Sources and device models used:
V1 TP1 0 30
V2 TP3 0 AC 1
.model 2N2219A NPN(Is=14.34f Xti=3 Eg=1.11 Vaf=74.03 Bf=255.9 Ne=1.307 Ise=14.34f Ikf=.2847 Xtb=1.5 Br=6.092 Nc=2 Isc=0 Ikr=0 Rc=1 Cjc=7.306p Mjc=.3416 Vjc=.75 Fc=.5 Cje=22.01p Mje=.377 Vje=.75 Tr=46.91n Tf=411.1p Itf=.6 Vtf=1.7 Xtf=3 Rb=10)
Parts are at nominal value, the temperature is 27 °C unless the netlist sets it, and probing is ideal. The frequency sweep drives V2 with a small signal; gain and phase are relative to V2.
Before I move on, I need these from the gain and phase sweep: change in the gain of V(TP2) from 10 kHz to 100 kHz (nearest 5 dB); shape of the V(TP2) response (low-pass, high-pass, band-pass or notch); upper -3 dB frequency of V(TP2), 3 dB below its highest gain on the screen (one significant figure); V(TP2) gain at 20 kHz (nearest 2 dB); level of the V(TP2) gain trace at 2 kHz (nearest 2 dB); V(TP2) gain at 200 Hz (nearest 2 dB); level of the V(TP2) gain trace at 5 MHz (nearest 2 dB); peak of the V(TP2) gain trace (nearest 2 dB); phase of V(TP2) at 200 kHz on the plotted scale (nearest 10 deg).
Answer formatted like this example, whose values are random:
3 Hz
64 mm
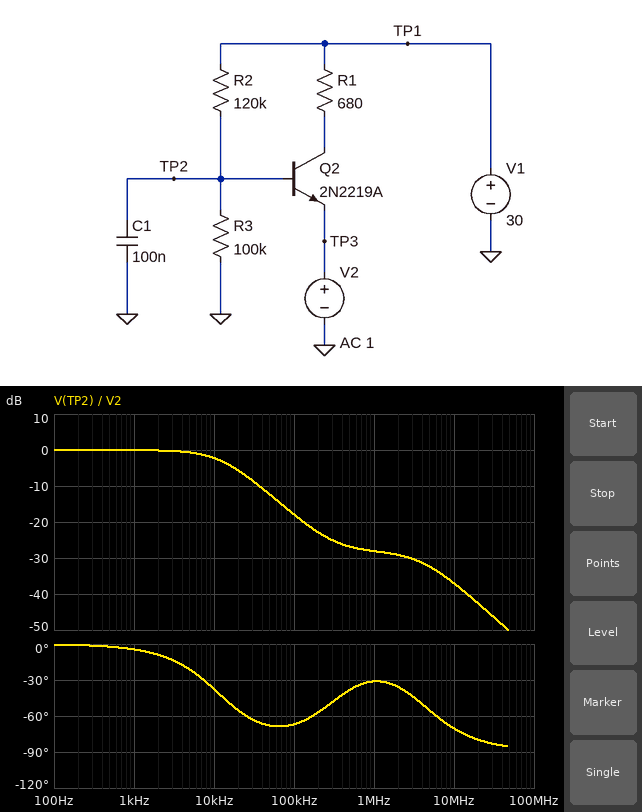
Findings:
-15 dB
low-pass
10 kHz
-6 dB
0 dB
0 dB
-32 dB
0 dB
-60 deg
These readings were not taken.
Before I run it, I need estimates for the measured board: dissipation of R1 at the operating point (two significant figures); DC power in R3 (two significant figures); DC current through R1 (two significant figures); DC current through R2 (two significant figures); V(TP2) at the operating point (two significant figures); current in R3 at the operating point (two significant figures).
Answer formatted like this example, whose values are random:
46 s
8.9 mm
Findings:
1.2 W
5.6 µW
41 mA
240 µA
750 mV
7.5 µA
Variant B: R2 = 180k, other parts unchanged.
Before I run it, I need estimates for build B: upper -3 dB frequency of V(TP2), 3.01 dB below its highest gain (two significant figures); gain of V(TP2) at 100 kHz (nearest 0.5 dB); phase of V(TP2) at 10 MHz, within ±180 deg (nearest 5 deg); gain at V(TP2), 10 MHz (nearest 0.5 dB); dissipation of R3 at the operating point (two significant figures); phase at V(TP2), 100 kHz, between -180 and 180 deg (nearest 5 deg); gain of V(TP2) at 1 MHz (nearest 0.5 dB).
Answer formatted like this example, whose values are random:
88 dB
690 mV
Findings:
8.4 kHz
-21.5 dB
-55 deg
-38.5 dB
5.4 µW
-70 deg
-33.0 dB
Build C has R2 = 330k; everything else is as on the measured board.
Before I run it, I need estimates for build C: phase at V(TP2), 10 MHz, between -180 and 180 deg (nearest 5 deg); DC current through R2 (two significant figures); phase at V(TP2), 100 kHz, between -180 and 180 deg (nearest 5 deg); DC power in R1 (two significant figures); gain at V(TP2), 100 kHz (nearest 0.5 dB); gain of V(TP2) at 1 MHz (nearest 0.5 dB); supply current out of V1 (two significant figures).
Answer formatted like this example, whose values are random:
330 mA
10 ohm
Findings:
-40 deg
89 µA
-75 deg
210 mW
-26.5 dB
-38.0 dB
18 mA
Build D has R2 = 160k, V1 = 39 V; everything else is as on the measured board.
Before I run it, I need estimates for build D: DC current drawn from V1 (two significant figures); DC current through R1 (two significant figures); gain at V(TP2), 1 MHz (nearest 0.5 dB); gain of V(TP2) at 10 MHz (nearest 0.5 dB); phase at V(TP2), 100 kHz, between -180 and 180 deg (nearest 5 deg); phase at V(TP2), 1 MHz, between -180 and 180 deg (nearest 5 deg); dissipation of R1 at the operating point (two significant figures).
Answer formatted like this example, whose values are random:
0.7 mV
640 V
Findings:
45 mA
44 mA
-31.0 dB
-37.5 dB
-70 deg
-35 deg
1.3 W
